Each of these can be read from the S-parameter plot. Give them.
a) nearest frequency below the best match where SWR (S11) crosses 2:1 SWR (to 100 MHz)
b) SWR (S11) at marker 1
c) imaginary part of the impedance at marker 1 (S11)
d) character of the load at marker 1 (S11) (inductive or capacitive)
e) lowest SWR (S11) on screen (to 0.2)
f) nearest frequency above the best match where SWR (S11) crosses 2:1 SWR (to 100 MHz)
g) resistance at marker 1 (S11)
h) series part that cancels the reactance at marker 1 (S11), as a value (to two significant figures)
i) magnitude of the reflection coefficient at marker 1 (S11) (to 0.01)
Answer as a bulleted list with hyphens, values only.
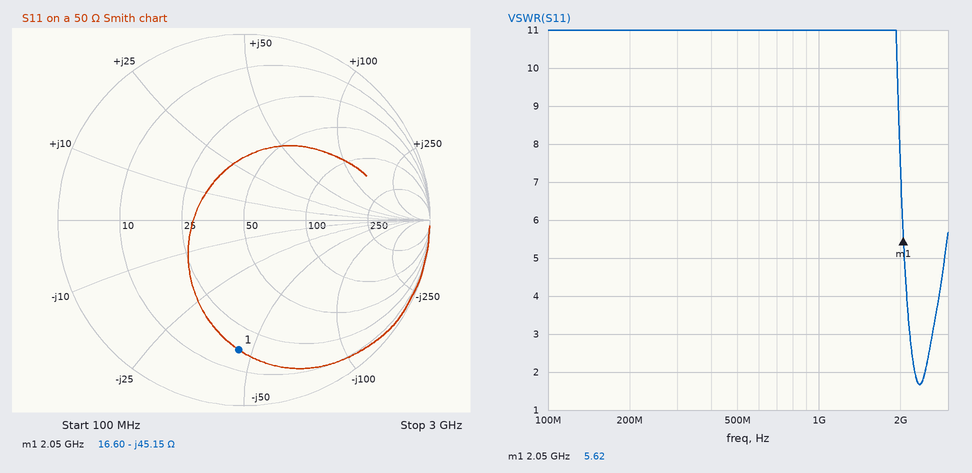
- 2.3 GHz
- 5.62
- -45.15 Ω
- capacitive
- 1.6
- 2.5 GHz
- 16.60 Ω
- 3.5 nH
- 0.70
